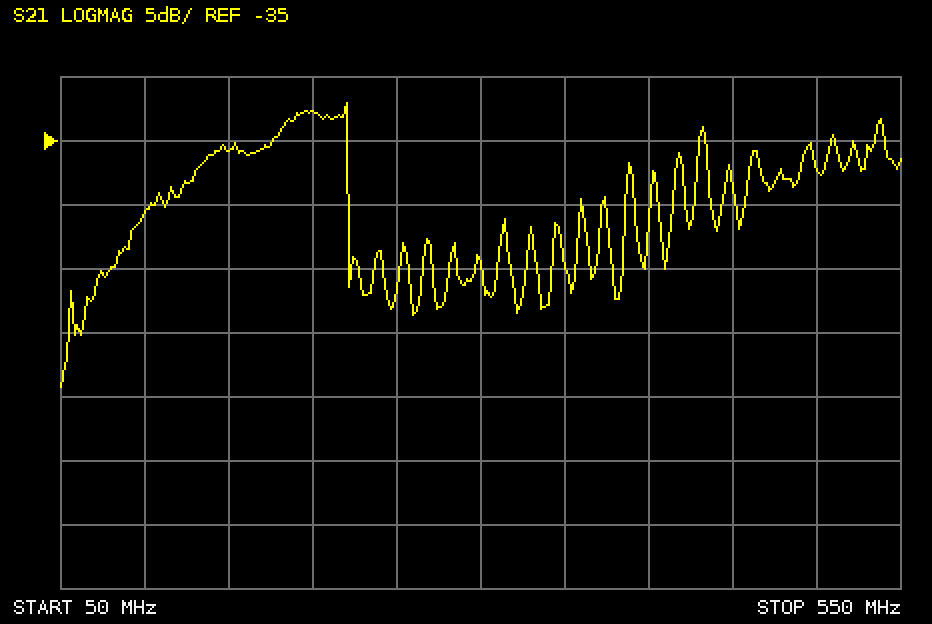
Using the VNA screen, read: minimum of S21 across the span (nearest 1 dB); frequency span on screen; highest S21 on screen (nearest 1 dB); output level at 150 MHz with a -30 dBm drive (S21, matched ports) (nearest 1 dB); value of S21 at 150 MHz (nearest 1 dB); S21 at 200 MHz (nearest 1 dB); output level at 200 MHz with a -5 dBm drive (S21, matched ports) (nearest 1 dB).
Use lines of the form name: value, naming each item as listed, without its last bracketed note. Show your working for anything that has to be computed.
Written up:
minimum of S21 across the span: -54 dB
frequency span on screen: 500 MHz
highest S21 on screen: -32 dB
output level at 150 MHz with a -30 dBm drive (S21, matched ports): -30 dBm + (-36 dB) = -66 dBm
value of S21 at 150 MHz: -36 dB
S21 at 200 MHz: -33 dB
output level at 200 MHz with a -5 dBm drive (S21, matched ports): -5 dBm + (-33 dB) = -38 dBm
